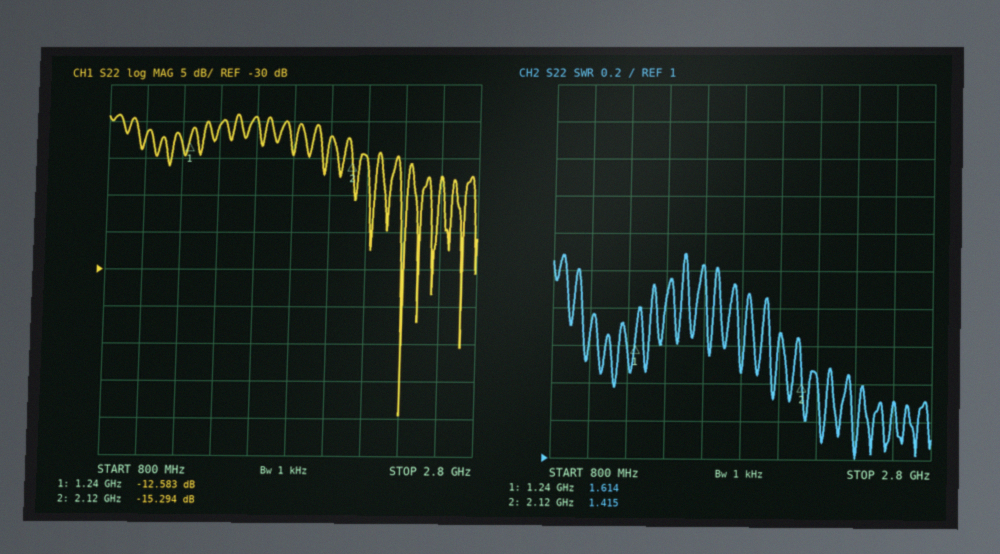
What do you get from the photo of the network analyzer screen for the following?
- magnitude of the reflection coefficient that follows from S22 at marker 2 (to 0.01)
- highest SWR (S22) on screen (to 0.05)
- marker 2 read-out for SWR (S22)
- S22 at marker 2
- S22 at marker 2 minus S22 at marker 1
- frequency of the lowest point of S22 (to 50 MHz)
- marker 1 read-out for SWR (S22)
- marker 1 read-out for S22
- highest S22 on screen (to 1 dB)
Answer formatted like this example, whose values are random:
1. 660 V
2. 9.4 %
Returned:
1. 0.17
2. 2.10
3. 1.415
4. -15.294 dB
5. -2.711 dB
6. 2.40 GHz
7. 1.614
8. -12.583 dB
9. -9 dB
